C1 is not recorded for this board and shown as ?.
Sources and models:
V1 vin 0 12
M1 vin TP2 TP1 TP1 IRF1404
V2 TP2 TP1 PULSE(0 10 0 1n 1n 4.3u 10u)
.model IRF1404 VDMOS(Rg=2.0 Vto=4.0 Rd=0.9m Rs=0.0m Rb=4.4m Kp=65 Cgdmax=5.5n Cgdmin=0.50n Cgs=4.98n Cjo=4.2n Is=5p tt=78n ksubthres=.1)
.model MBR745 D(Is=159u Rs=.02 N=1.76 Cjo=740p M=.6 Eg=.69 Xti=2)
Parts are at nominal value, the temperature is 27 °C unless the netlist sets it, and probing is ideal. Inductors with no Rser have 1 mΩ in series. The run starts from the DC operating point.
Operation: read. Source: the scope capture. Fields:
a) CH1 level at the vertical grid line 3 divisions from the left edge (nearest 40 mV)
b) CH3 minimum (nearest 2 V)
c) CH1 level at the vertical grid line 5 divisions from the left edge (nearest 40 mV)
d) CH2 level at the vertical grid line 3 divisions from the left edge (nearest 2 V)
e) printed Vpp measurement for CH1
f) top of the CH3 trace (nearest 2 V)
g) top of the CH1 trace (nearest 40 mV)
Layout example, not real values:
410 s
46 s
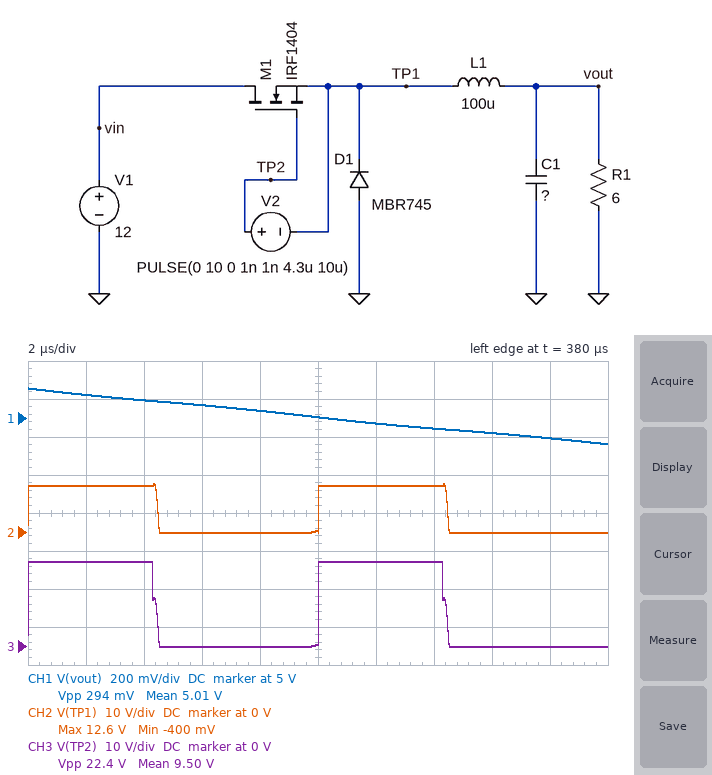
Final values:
5.08 V
0 V
5.00 V
0 V
294 mV
22 V
5.16 V
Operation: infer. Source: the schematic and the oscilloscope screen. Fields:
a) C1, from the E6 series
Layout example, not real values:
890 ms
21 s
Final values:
47 µF
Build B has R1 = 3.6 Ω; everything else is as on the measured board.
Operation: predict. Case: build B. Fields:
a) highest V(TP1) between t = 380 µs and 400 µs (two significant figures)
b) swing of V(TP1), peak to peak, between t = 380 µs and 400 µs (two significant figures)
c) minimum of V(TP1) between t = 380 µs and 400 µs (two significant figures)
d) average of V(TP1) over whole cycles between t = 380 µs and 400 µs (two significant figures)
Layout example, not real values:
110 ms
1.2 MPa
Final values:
12 V
13 V
-420 mV
5.0 V
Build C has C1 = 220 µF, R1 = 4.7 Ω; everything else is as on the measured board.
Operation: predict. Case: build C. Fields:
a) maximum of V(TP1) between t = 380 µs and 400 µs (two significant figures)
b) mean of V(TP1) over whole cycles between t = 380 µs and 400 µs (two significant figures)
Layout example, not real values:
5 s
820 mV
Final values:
12 V
4.9 V
